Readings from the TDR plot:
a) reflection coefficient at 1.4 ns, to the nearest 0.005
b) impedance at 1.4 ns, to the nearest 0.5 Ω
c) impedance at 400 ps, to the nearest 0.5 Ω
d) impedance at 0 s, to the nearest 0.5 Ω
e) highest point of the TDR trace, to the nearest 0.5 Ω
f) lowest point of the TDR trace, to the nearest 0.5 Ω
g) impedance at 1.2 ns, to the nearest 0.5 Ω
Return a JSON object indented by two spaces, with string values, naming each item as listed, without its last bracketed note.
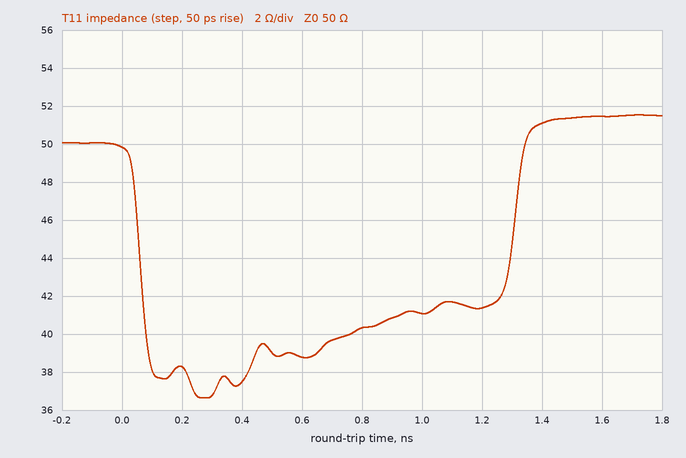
{
  "reflection coefficient at 1.4 ns, to the nearest 0.005": "+0.010",
  "impedance at 1.4 ns, to the nearest 0.5 Ω": "51.0 Ω",
  "impedance at 400 ps, to the nearest 0.5 Ω": "37.5 Ω",
  "impedance at 0 s, to the nearest 0.5 Ω": "50.0 Ω",
  "highest point of the TDR trace, to the nearest 0.5 Ω": "51.5 Ω",
  "lowest point of the TDR trace, to the nearest 0.5 Ω": "36.5 Ω",
  "impedance at 1.2 ns, to the nearest 0.5 Ω": "41.5 Ω"
}
